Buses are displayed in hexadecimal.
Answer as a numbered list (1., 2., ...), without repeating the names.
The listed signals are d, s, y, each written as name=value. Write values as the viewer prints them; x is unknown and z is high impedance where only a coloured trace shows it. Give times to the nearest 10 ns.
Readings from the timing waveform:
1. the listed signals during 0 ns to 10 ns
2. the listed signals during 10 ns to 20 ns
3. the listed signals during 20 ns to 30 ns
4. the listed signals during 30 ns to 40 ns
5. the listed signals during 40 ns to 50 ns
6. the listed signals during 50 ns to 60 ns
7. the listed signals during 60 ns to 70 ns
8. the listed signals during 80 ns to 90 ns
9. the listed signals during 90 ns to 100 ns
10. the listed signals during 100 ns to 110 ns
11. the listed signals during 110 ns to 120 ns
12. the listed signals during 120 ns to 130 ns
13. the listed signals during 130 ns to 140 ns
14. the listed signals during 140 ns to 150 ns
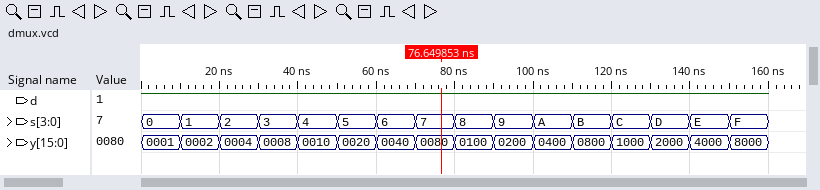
1. d=1, s=0, y=0001
2. d=1, s=1, y=0002
3. d=1, s=2, y=0004
4. d=1, s=3, y=0008
5. d=1, s=4, y=0010
6. d=1, s=5, y=0020
7. d=1, s=6, y=0040
8. d=1, s=8, y=0100
9. d=1, s=9, y=0200
10. d=1, s=A, y=0400
11. d=1, s=B, y=0800
12. d=1, s=C, y=1000
13. d=1, s=D, y=2000
14. d=1, s=E, y=4000
